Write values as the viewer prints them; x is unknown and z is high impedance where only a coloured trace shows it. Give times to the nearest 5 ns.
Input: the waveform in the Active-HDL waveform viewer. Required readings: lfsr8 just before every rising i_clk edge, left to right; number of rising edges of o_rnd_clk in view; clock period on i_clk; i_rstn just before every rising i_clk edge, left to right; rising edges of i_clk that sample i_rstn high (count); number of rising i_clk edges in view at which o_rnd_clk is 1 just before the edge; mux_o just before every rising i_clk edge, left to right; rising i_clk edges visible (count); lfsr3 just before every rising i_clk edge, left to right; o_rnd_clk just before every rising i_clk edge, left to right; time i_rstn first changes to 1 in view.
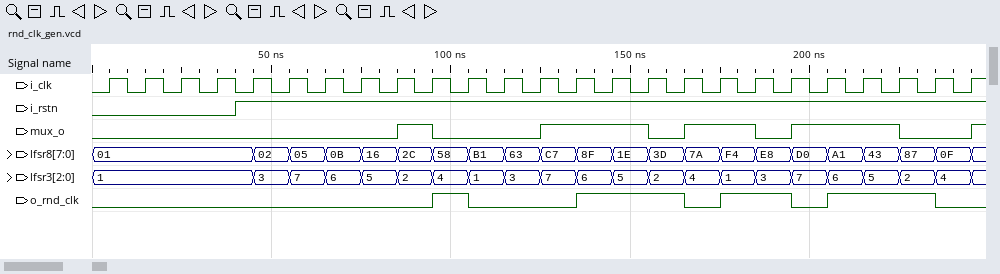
01, 01, 01, 01, 01, 02, 05, 0B, 16, 2C, 58, B1, 63, C7, 8F, 1E, 3D, 7A, F4, E8, D0, A1, 43, 87, 0F
4
10 ns
0 0 0 0 1 1 1 1 1 1 1 1 1 1 1 1 1 1 1 1 1 1 1 1 1
21
9
0 0 0 0 0 0 0 0 0 1 0 0 0 1 1 1 0 1 1 0 1 1 1 0 0
25
1, 1, 1, 1, 1, 3, 7, 6, 5, 2, 4, 1, 3, 7, 6, 5, 2, 4, 1, 3, 7, 6, 5, 2, 4
0 0 0 0 0 0 0 0 0 0 1 0 0 0 1 1 1 0 1 1 0 1 1 1 0
40 ns
